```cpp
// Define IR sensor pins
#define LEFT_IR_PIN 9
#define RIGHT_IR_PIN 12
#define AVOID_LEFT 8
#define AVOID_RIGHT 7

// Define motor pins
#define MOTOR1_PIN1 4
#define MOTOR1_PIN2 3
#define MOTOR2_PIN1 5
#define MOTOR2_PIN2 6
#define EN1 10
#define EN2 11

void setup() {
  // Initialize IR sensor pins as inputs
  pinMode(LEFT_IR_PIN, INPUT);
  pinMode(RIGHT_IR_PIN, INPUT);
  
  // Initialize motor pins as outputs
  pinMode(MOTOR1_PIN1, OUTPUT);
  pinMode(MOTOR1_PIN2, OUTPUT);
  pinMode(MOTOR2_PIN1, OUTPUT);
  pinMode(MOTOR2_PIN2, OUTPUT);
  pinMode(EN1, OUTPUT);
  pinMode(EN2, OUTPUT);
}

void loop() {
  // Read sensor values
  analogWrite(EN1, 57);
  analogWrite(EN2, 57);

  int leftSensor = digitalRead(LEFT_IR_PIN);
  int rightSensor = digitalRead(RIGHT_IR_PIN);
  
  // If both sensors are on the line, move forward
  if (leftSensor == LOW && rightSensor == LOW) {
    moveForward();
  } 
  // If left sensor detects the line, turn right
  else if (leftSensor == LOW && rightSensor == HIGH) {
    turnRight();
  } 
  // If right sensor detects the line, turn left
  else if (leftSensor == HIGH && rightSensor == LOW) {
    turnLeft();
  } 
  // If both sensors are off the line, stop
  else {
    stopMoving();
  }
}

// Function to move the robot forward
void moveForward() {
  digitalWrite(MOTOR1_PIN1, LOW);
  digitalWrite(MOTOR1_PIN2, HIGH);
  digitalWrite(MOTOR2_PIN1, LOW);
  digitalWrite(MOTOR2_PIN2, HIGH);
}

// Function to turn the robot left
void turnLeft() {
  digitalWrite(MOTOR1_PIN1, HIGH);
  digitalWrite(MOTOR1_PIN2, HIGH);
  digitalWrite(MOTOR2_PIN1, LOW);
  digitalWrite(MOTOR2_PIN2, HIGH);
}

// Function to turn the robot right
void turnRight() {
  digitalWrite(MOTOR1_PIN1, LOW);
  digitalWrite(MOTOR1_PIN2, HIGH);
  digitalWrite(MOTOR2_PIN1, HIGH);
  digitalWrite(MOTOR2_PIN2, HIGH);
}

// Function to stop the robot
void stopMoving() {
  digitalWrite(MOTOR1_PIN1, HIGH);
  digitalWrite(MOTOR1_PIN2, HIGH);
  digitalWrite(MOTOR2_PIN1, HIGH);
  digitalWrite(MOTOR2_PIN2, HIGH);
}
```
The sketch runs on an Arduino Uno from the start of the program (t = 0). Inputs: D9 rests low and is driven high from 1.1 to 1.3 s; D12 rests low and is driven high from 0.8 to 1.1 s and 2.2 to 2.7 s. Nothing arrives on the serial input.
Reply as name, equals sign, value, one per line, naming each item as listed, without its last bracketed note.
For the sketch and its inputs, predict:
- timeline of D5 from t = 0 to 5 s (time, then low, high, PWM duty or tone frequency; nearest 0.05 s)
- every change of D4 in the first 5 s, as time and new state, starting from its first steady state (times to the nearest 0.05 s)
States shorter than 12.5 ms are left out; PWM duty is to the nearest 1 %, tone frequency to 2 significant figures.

timeline of D5 from t = 0 to 5 s = 0 s low; 0.8 s high; 1.1 s low; 2.2 s high; 2.7 s low
every change of D4 in the first 5 s, as time and new state, starting from its first steady state = 0 s low; 1.1 s high; 1.3 s low
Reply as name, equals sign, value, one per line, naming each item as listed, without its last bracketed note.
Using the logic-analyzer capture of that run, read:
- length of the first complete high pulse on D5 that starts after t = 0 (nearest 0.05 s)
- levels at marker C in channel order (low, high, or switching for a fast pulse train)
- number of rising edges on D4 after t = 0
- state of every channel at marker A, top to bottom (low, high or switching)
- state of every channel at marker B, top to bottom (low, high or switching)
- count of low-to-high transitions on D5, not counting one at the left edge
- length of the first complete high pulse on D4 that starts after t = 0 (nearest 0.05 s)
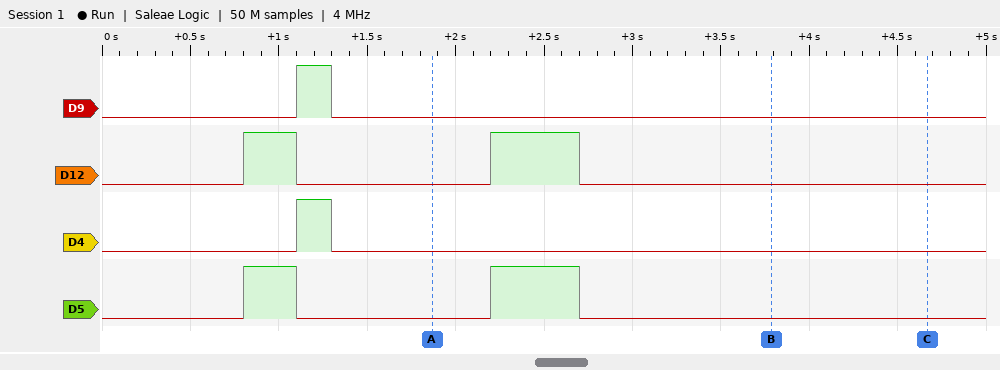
length of the first complete high pulse on D5 that starts after t = 0 = 0.30 s
levels at marker C in channel order = D9 low, D12 low, D4 low, D5 low
number of rising edges on D4 after t = 0 = 1
state of every channel at marker A, top to bottom = D9 low, D12 low, D4 low, D5 low
state of every channel at marker B, top to bottom = D9 low, D12 low, D4 low, D5 low
count of low-to-high transitions on D5, not counting one at the left edge = 2
length of the first complete high pulse on D4 that starts after t = 0 = 0.20 s
